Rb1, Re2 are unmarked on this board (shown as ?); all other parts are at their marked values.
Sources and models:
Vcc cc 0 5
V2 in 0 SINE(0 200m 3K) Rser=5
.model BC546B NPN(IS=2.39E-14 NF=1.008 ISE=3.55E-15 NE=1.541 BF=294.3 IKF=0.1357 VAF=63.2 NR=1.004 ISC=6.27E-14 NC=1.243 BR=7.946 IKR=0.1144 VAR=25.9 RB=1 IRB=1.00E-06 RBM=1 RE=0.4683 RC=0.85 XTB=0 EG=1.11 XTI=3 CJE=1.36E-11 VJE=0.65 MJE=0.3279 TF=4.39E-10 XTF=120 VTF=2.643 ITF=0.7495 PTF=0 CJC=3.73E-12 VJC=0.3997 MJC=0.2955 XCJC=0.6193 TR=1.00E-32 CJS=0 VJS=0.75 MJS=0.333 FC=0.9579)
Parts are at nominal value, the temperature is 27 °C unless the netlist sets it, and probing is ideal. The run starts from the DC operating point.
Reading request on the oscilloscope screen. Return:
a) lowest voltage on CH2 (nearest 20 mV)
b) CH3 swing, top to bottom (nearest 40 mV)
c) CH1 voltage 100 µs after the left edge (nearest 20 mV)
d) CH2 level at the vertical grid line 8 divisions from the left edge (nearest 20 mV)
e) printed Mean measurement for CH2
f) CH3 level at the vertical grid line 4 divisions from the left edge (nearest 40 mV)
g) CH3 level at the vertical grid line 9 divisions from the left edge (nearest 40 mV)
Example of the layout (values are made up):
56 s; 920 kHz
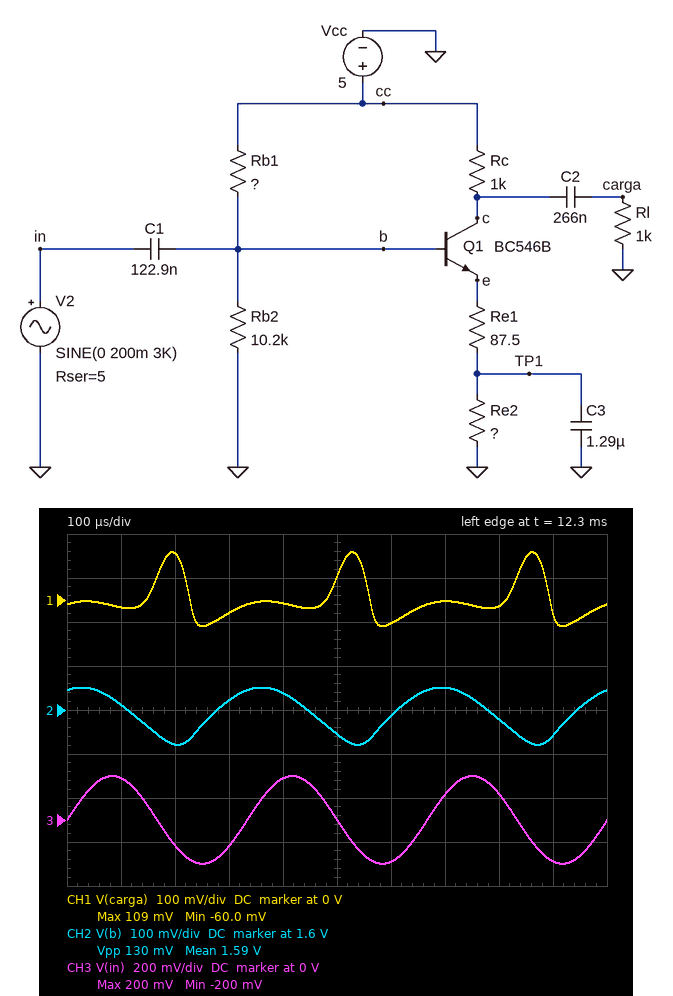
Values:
1.52 V; 400 mV; -20 mV; 1.58 V; 1.59 V; 200 mV; -200 mV
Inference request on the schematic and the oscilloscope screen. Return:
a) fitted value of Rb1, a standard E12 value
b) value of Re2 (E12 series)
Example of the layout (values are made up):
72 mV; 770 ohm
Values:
6.8 kΩ; 120 Ω
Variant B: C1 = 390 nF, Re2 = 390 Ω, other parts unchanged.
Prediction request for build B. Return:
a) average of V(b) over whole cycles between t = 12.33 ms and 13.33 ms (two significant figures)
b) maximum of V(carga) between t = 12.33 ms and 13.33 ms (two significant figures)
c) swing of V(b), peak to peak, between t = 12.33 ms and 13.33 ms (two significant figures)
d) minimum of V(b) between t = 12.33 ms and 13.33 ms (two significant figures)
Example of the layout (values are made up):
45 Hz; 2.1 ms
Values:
2.2 V; 680 mV; 350 mV; 2.0 V
